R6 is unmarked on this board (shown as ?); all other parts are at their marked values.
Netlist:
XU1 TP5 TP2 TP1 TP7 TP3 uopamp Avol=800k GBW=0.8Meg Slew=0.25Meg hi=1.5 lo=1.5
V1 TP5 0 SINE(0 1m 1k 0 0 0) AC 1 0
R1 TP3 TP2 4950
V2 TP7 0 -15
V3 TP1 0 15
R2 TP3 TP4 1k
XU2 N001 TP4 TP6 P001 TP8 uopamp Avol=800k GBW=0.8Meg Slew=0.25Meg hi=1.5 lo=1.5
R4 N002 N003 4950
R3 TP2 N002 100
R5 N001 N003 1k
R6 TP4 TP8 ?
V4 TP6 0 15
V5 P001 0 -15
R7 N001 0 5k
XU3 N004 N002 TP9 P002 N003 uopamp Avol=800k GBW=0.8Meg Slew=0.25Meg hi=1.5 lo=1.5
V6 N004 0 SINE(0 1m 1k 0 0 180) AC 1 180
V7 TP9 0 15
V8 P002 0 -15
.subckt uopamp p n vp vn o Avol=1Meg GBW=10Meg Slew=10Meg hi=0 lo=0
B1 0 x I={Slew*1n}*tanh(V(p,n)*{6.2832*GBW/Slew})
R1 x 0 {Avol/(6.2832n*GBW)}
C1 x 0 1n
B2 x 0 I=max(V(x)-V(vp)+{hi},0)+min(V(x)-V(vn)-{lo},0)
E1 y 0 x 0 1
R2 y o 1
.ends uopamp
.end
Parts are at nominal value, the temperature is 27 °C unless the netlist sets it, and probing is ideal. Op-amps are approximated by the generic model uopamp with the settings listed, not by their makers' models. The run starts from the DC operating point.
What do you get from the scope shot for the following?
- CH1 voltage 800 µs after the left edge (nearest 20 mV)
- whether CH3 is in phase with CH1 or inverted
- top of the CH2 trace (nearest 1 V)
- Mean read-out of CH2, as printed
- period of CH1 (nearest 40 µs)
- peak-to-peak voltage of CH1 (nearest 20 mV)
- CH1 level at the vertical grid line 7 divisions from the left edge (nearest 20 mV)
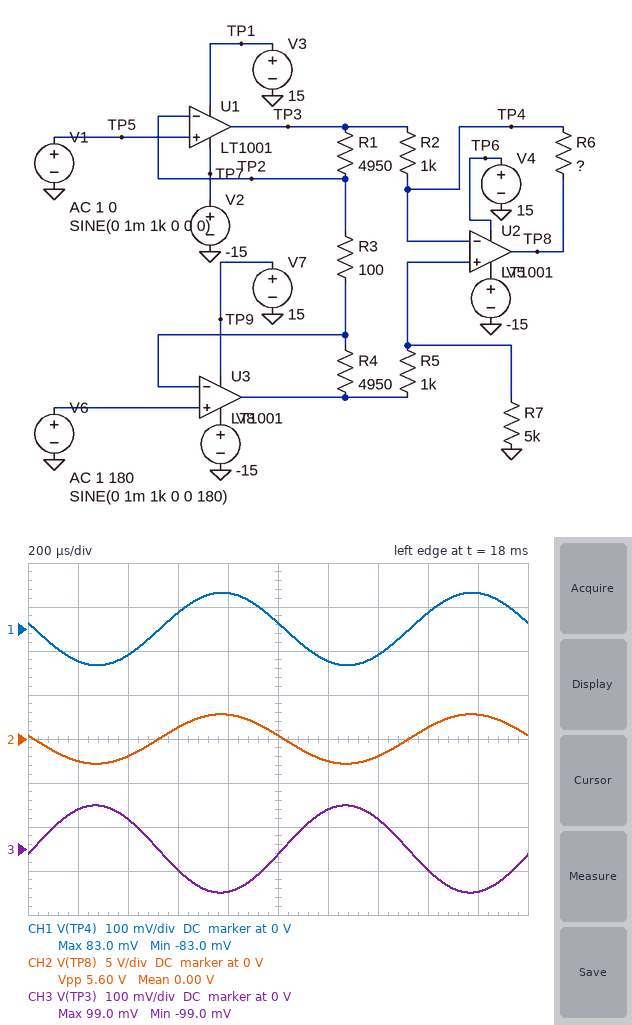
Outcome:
80 mV
inverted
3 V
0.00 V
1.00 ms
160 mV
-60 mV
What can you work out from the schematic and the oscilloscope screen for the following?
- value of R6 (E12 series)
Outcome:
15 kΩ
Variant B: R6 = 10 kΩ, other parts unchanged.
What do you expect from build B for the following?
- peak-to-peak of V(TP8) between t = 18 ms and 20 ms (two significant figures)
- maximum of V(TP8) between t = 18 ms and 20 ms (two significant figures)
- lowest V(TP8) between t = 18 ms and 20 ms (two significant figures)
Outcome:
3.8 V
1.9 V
-1.9 V
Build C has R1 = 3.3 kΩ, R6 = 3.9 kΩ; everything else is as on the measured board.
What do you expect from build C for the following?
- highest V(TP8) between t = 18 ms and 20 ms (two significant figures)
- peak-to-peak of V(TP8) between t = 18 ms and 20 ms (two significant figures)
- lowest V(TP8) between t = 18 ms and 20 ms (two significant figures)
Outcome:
670 mV
1.3 V
-670 mV
